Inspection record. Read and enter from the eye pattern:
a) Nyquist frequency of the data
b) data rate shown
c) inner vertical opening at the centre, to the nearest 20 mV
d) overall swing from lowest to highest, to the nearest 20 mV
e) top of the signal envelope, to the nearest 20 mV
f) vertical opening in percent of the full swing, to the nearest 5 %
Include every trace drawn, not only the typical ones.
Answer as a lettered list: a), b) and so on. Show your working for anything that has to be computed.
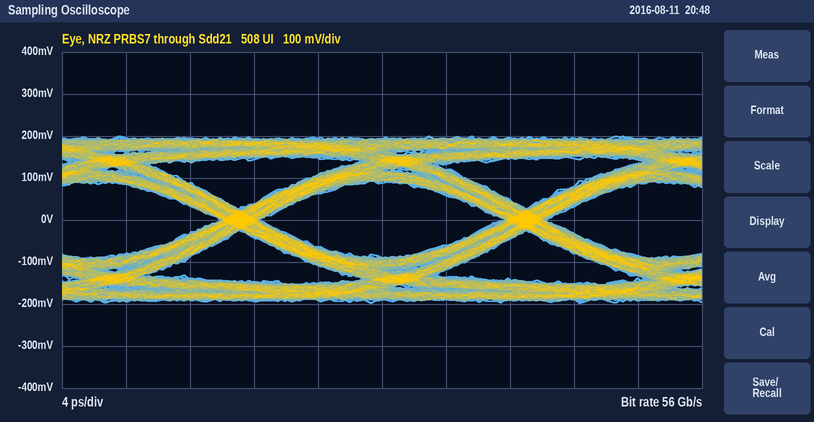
a) 28 GHz
b) 56 Gb/s
c) 180 mV
d) 400 mV
e) 200 mV
f) 180 mV / 400 mV ≈ 45 %
